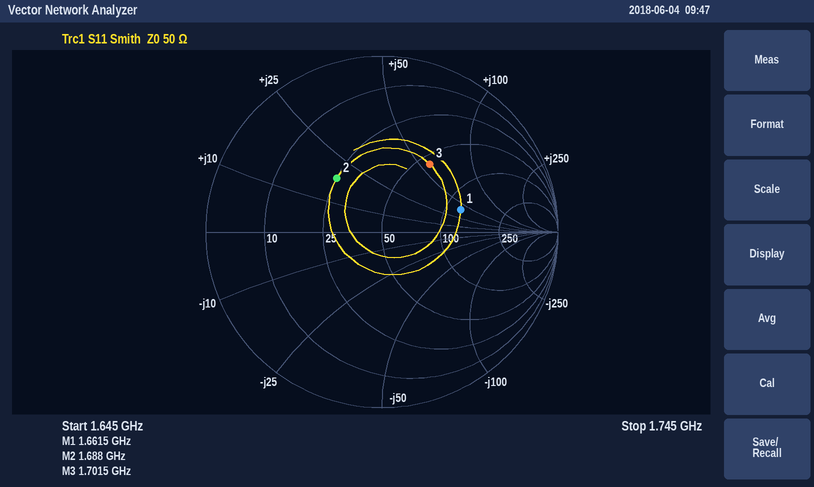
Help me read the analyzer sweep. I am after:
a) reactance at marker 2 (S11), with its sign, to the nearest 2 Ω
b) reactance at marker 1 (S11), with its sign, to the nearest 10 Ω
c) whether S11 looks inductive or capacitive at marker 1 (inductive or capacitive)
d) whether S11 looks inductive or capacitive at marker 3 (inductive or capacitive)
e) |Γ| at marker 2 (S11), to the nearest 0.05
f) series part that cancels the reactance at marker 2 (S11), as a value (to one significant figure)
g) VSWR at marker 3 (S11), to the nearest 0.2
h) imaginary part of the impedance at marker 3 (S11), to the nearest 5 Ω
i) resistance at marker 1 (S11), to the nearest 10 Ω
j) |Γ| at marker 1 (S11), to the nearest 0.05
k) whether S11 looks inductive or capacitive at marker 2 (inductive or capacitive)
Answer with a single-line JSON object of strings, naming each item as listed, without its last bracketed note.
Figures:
{"reactance at marker 2 (S11), with its sign, to the nearest 2 Ω": "+18 Ω", "reactance at marker 1 (S11), with its sign, to the nearest 10 Ω": "+40 Ω", "whether S11 looks inductive or capacitive at marker 1": "inductive", "whether S11 looks inductive or capacitive at marker 3": "inductive", "|Γ| at marker 2 (S11), to the nearest 0.05": "0.40", "series part that cancels the reactance at marker 2 (S11), as a value": "5 pF", "VSWR at marker 3 (S11), to the nearest 0.2": "2.8", "imaginary part of the impedance at marker 3 (S11), to the nearest 5 Ω": "+55 Ω", "resistance at marker 1 (S11), to the nearest 10 Ω": "120 Ω", "|Γ| at marker 1 (S11), to the nearest 0.05": "0.45", "whether S11 looks inductive or capacitive at marker 2": "inductive"}
